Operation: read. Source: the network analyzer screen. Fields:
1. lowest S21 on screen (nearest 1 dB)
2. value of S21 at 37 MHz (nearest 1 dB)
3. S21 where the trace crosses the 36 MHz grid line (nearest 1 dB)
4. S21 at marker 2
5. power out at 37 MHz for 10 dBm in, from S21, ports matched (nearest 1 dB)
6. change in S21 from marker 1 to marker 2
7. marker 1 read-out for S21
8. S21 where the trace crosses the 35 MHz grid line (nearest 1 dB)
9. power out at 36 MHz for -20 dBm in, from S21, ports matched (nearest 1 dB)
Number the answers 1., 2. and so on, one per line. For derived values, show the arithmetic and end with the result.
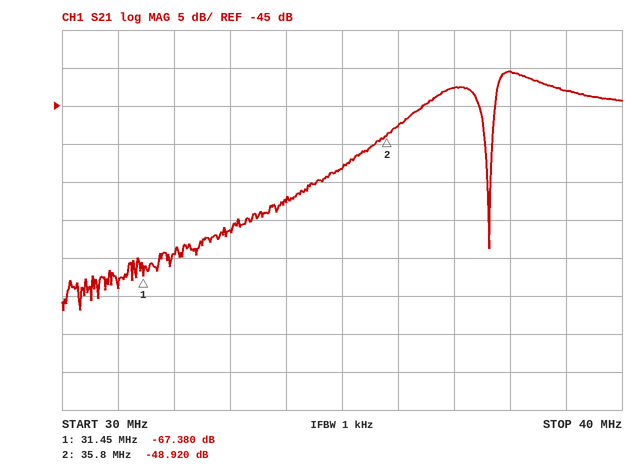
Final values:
1. -72 dB
2. -43 dB
3. -48 dB
4. -48.920 dB
5. 10 dBm + (-43 dB) = -33 dBm
6. -48.92 − (-67.38) = 18.460 dB
7. -67.380 dB
8. -53 dB
9. -20 dBm + (-48 dB) = -68 dBm
